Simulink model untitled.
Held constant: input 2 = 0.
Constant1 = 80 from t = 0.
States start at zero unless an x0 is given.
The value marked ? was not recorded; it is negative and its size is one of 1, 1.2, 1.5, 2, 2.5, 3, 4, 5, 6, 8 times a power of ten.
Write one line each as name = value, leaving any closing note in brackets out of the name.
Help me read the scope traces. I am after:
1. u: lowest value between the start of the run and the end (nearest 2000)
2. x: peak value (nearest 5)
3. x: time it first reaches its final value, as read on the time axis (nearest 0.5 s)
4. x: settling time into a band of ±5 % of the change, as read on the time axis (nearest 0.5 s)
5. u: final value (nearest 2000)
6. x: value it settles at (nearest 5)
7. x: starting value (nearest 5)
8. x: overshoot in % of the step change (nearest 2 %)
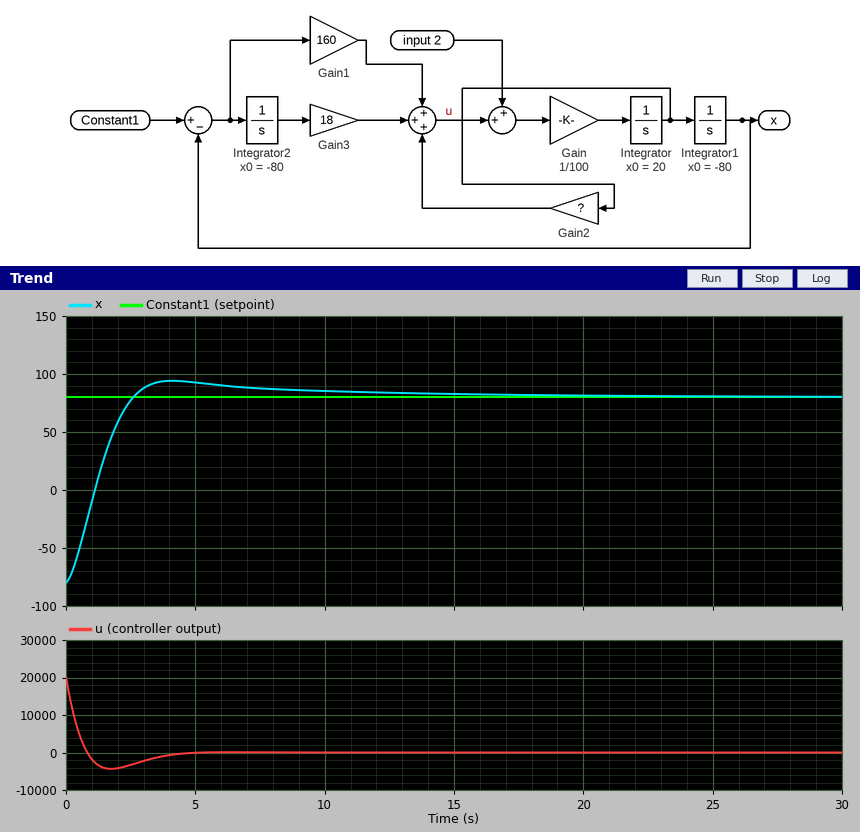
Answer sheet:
u: lowest value between the start of the run and the end = -4000
x: peak value = 95
x: time it first reaches its final value, as read on the time axis = 2.5 s
x: settling time into a band of ±5 % of the change, as read on the time axis = 7.0 s
u: final value = 0
x: value it settles at = 80
x: starting value = -80
x: overshoot in % of the step change = 8 %
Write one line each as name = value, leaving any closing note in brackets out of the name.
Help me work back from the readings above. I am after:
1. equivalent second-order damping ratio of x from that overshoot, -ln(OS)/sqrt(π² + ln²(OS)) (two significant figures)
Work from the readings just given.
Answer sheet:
equivalent second-order damping ratio of x from that overshoot, -ln(OS)/sqrt(π² + ln²(OS)) = 0.63
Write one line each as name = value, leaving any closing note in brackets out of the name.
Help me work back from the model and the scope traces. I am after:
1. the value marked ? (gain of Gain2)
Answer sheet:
the value marked ? = -200
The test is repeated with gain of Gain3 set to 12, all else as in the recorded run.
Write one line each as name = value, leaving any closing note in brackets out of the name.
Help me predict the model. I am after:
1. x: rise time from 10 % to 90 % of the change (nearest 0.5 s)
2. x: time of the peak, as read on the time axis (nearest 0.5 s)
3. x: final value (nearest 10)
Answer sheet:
x: rise time from 10 % to 90 % of the change = 2.0 s
x: time of the peak, as read on the time axis = 4.0 s
x: final value = 80
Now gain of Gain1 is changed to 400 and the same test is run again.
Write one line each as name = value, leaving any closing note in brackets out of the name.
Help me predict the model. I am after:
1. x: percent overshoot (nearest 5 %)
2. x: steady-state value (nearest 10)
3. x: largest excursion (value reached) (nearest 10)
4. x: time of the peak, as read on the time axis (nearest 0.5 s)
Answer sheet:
x: percent overshoot = 15 %
x: steady-state value = 80
x: largest excursion (value reached) = 110
x: time of the peak, as read on the time axis = 2.0 s
